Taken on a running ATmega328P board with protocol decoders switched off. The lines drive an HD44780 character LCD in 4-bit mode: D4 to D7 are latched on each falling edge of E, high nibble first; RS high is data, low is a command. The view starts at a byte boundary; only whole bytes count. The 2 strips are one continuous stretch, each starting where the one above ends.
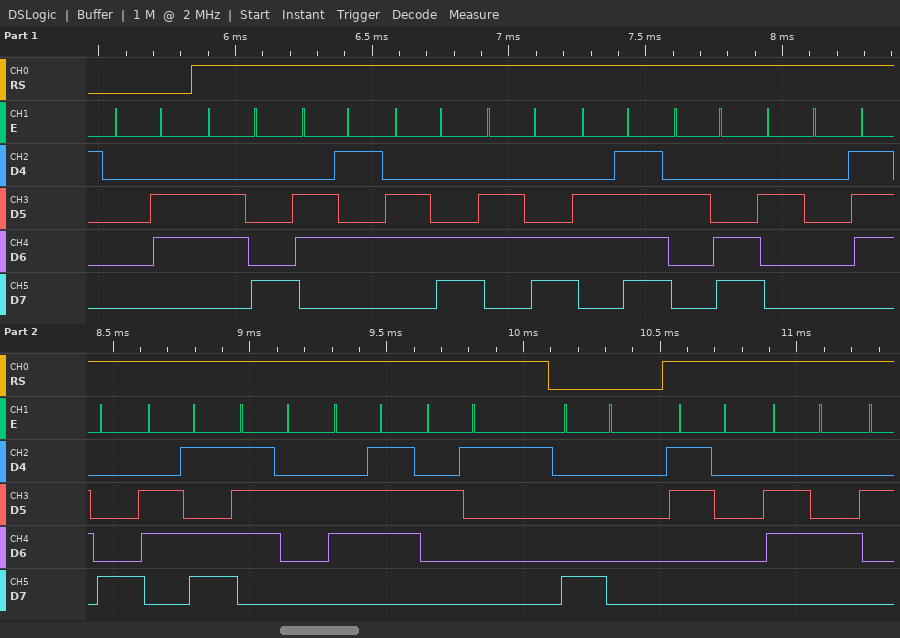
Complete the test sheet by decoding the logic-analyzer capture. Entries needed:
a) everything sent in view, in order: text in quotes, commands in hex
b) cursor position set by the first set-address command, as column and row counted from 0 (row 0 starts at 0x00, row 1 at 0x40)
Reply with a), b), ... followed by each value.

a) 0x06 "hello, xmrg!" 0x80 "0d"
b) column 0, row 0
